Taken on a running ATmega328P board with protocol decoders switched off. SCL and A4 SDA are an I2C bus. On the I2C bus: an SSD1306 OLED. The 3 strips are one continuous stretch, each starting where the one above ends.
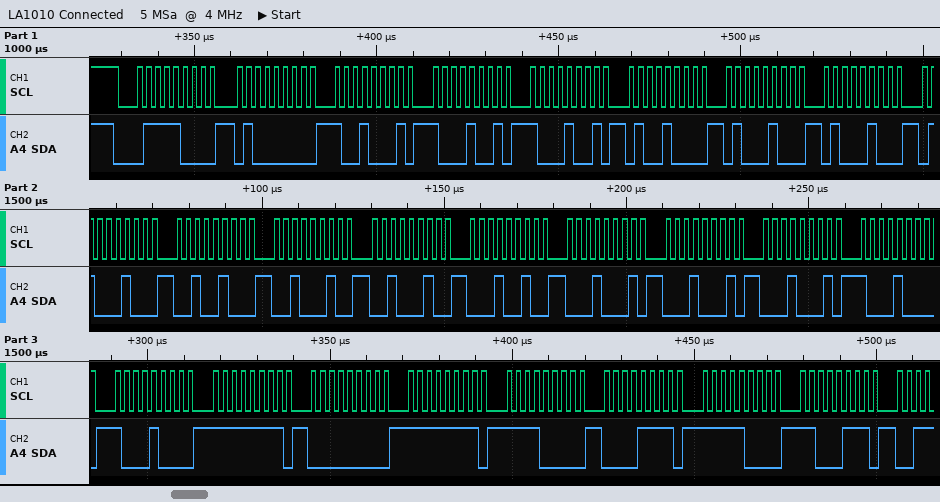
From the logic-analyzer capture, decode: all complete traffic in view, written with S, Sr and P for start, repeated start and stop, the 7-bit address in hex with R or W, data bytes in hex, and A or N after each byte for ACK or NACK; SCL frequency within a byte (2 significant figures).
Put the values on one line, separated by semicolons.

S 3CW A 40 A 91 A 89 A 89 A 48 A 44 A 44 A 44 A 24 A 22 A 22 A 12 A 11 A 11 A 11 A 88 A 88 A FF A 00 A FF A F0 A 0F A F8 A C7 A; 400 kHz
